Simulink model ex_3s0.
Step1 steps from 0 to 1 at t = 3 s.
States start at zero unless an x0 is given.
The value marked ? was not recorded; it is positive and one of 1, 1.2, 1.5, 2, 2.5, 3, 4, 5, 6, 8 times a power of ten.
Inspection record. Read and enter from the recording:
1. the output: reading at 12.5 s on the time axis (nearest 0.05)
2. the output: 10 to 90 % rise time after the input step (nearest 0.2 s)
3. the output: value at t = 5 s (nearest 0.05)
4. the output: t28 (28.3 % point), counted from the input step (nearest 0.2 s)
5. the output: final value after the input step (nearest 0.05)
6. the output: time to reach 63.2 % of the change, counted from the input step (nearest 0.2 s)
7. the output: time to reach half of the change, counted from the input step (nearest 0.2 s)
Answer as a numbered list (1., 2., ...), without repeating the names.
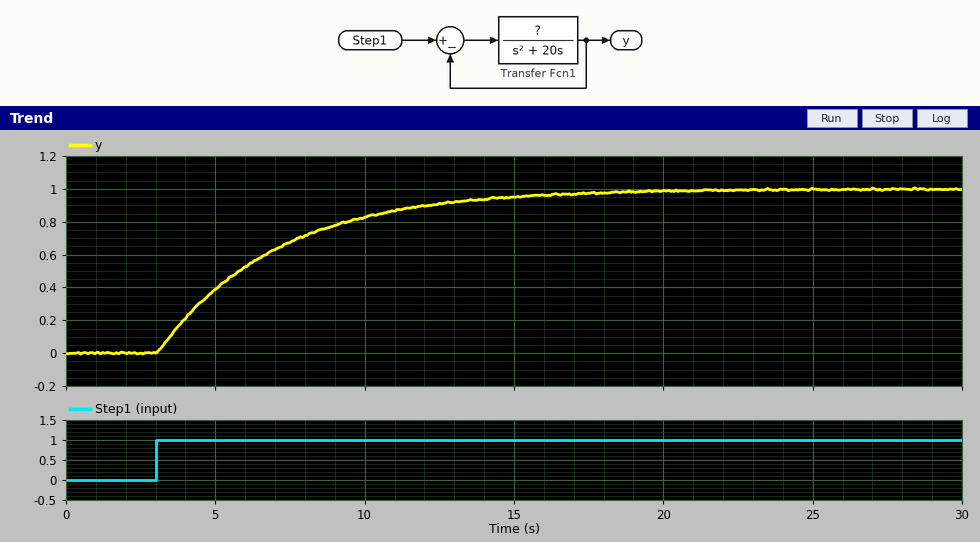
1. 0.90
2. 8.6 s
3. 0.40
4. 1.4 s
5. 1.00
6. 4.0 s
7. 2.8 s
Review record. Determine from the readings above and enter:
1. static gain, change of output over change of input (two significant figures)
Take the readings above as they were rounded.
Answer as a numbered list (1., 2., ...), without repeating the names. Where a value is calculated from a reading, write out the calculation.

1. (1 - 0) / (1 - 0) = 1.0
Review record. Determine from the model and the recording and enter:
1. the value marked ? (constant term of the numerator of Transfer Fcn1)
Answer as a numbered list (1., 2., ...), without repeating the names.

1. 5
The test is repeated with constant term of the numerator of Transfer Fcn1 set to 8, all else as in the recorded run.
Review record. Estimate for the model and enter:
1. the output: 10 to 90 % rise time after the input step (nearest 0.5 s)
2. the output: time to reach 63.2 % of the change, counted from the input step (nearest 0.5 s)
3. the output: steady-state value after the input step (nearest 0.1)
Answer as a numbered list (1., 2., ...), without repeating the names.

1. 5.5 s
2. 2.5 s
3. 1.0
